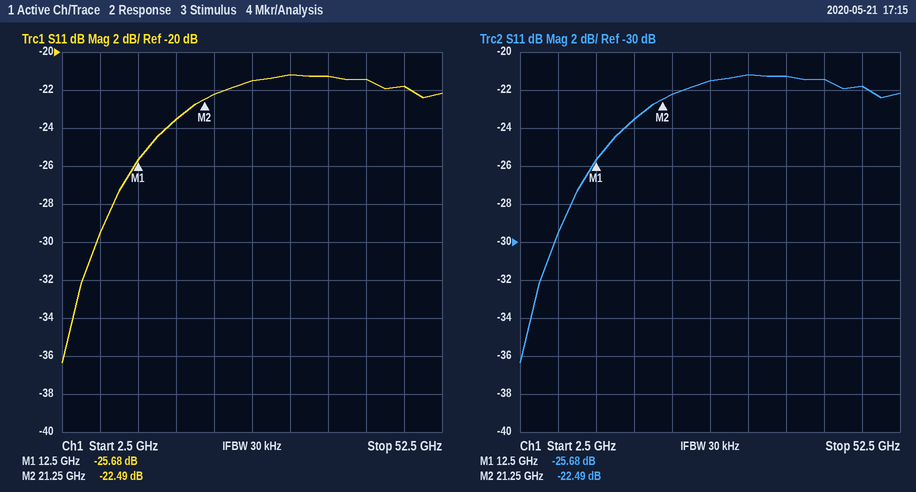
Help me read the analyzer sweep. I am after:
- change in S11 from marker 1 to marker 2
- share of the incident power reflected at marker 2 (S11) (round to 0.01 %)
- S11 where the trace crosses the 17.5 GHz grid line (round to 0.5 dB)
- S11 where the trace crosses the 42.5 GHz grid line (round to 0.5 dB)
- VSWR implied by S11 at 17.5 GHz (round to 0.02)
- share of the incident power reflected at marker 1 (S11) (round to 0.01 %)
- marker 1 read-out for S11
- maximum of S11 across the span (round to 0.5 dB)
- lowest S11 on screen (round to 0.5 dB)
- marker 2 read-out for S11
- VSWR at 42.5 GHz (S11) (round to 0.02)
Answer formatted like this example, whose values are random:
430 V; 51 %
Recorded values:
3.19 dB; 0.56 %; -23.5 dB; -21.5 dB; 1.14; 0.27 %; -25.68 dB; -21.0 dB; -36.5 dB; -22.49 dB; 1.18
